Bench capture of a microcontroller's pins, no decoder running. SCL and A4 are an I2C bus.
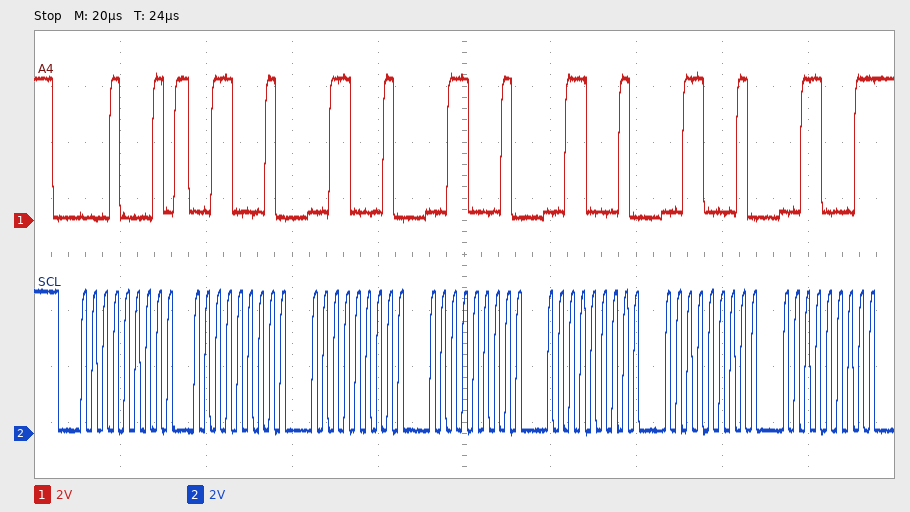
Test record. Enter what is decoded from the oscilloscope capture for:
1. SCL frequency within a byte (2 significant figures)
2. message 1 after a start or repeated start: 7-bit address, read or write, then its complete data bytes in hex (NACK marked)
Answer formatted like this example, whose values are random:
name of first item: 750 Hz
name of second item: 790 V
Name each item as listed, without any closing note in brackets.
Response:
SCL frequency within a byte: 400 kHz
message 1 after a start or repeated start: 7-bit address, read or write, then its complete data bytes in hex: 0x08 read: 31 31 31 31 31 31 NACK
